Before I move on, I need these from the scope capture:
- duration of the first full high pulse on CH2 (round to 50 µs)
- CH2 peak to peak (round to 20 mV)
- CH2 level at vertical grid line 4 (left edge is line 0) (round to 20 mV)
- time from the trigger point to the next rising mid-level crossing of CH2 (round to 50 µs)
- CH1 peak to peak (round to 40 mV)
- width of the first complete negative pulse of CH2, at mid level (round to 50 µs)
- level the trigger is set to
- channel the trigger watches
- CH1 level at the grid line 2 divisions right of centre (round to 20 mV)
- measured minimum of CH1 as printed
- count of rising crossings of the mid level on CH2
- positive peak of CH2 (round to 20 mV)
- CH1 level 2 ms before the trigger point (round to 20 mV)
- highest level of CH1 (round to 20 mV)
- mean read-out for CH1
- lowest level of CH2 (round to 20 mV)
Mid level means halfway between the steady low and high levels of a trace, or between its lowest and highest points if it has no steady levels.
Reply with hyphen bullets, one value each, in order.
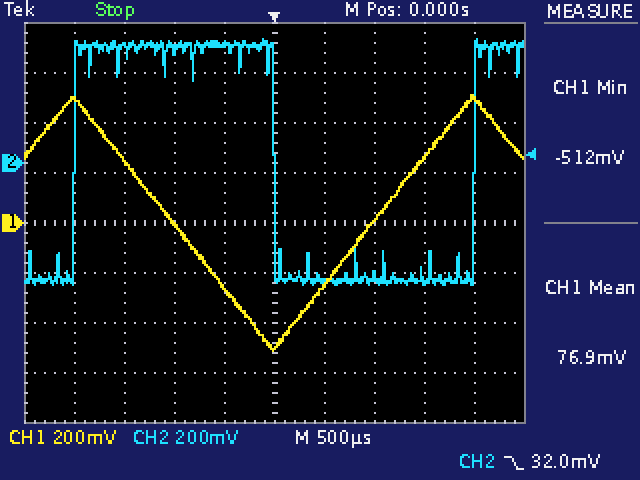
- 2.00 ms
- 980 mV
- 480 mV
- 2.00 ms
- 1.04 V
- 2.00 ms
- 32.0 mV
- CH2
- 20 mV
- -512 mV
- 2
- 500 mV
- 500 mV
- 520 mV
- 76.9 mV
- -480 mV
